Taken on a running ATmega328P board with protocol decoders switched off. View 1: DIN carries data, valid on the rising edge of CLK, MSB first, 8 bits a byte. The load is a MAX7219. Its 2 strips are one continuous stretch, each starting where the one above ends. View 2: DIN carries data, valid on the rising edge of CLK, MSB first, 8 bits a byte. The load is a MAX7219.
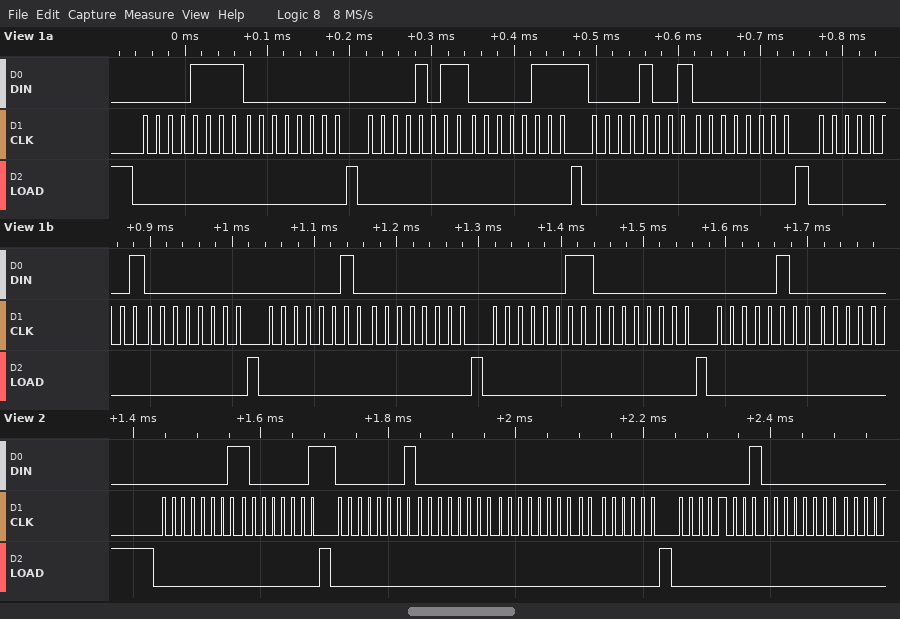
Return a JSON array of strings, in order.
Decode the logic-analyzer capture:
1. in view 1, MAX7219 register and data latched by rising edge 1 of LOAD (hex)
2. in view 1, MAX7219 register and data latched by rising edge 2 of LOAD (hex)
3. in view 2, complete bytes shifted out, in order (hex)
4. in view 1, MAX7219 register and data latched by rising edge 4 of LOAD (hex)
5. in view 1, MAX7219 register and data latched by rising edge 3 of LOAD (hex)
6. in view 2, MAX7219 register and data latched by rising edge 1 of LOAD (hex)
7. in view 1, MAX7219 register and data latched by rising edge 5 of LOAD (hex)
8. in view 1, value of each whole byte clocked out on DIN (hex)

["register 0xF, data 0x00", "register 0xB, data 0x07", "01 81 01 00 00 00 01 00", "register 0x1, data 0x00", "register 0x9, data 0x00", "register 0x1, data 0x81", "register 0x2, data 0x00", "0F 00 0B 07 09 00 01 00 02 00 03 00 04"]
